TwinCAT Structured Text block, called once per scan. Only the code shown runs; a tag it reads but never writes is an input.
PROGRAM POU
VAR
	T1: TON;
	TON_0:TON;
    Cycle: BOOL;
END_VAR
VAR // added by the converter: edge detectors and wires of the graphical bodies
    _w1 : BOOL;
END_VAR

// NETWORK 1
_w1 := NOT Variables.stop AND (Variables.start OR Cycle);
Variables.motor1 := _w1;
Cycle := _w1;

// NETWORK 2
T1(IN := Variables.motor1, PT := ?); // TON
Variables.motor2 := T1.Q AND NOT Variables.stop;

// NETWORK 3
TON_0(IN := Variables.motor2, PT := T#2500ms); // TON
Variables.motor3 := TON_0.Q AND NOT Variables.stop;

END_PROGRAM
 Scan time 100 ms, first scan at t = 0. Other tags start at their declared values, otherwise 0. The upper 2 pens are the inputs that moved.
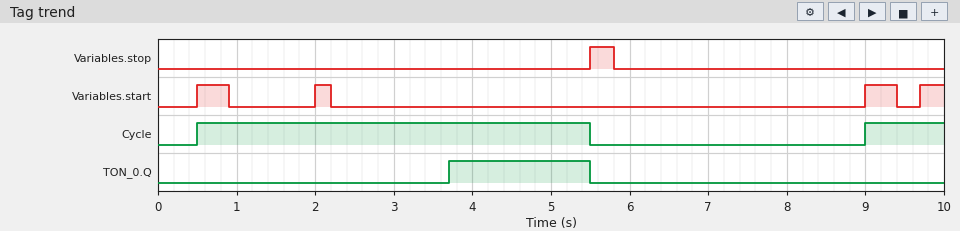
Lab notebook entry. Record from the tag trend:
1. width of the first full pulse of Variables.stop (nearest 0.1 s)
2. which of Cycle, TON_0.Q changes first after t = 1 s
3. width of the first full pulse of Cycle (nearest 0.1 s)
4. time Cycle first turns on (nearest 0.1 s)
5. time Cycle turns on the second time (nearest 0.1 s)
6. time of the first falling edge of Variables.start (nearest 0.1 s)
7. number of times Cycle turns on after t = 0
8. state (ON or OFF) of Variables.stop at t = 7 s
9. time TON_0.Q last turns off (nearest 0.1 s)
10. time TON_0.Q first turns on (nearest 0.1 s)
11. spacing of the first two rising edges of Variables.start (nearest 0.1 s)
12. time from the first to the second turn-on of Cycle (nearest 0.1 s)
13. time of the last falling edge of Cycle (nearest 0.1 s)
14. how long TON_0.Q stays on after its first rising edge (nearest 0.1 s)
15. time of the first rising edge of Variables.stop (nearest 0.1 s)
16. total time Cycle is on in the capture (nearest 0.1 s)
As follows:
0.3 s
TON_0.Q
5.0 s
0.5 s
9.0 s
0.9 s
2
OFF
5.5 s
3.7 s
1.5 s
8.5 s
5.5 s
1.8 s
5.5 s
6.0 s
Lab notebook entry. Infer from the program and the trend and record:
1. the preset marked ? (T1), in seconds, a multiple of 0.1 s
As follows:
0.7 s
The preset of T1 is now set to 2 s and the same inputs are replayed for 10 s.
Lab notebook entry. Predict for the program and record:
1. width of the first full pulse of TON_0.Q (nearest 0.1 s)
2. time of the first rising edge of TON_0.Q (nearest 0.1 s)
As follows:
0.5 s
5.0 s
